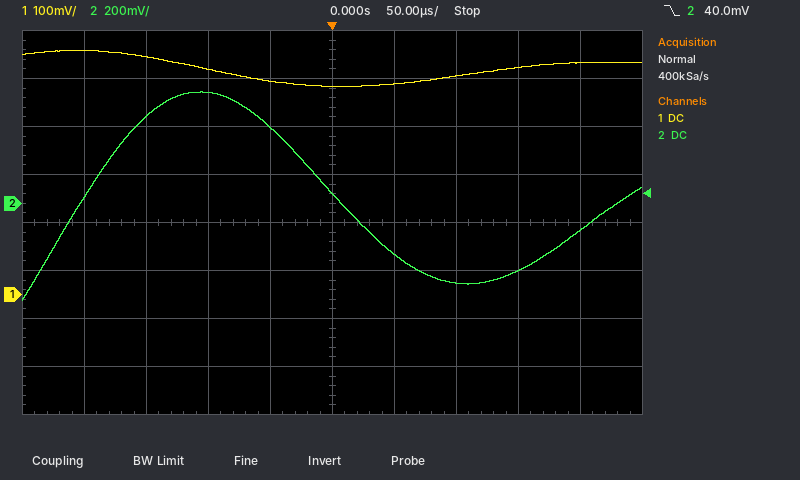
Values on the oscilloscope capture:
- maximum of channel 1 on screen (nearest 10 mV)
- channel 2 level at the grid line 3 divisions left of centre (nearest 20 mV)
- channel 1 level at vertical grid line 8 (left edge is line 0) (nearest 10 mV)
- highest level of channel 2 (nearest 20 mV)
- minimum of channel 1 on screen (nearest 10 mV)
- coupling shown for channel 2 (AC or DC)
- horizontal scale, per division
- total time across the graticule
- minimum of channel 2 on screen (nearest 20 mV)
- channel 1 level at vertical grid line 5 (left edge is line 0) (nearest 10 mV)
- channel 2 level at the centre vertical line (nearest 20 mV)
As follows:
510 mV
360 mV
470 mV
460 mV
430 mV
DC
50 µs
500 µs
-400 mV
430 mV
40 mV
